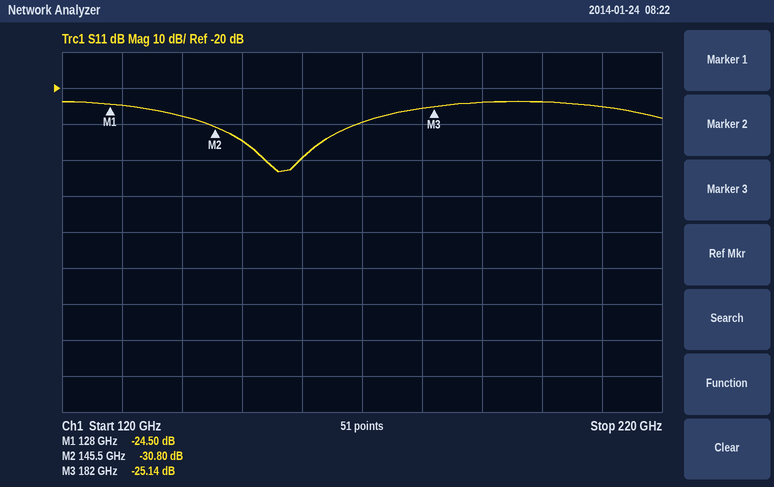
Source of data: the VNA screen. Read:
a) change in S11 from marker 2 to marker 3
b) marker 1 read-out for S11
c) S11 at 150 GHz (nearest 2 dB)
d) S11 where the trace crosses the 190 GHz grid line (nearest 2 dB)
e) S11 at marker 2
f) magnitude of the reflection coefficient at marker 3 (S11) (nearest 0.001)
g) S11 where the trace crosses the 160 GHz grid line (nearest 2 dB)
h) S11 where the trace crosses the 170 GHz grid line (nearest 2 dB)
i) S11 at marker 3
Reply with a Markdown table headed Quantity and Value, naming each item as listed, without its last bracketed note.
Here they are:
| Quantity | Value |
|---|---|
| change in S11 from marker 2 to marker 3 | 5.66 dB |
| marker 1 read-out for S11 | -24.50 dB |
| S11 at 150 GHz | -34 dB |
| S11 where the trace crosses the 190 GHz grid line | -24 dB |
| S11 at marker 2 | -30.80 dB |
| magnitude of the reflection coefficient at marker 3 (S11) | 0.055 |
| S11 where the trace crosses the 160 GHz grid line | -40 dB |
| S11 where the trace crosses the 170 GHz grid line | -30 dB |
| S11 at marker 3 | -25.14 dB |
